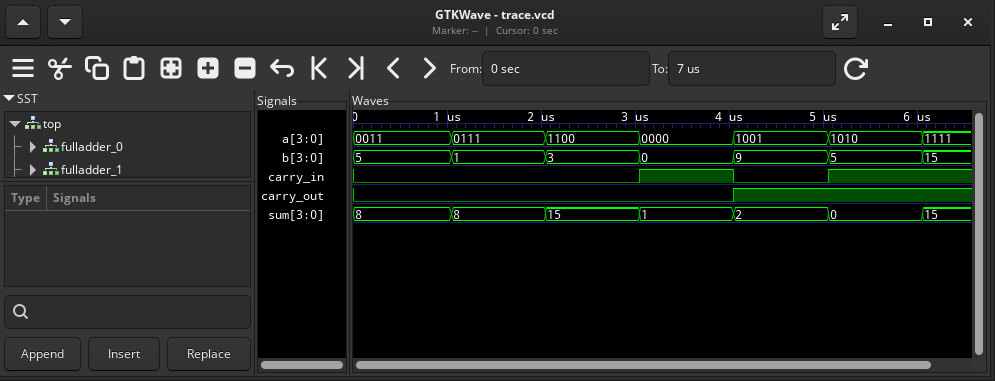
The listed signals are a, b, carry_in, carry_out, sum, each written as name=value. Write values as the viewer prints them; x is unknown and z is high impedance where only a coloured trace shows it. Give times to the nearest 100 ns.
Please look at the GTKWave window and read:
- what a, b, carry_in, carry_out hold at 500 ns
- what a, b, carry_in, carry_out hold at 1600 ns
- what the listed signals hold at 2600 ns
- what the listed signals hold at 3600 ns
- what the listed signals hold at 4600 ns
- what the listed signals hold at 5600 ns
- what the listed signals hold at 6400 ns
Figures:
a=0011, b=5, carry_in=0, carry_out=0
a=0111, b=1, carry_in=0, carry_out=0
a=1100, b=3, carry_in=0, carry_out=0, sum=15
a=0000, b=0, carry_in=1, carry_out=0, sum=1
a=1001, b=9, carry_in=0, carry_out=1, sum=2
a=1010, b=5, carry_in=1, carry_out=1, sum=0
a=1111, b=15, carry_in=1, carry_out=1, sum=15
